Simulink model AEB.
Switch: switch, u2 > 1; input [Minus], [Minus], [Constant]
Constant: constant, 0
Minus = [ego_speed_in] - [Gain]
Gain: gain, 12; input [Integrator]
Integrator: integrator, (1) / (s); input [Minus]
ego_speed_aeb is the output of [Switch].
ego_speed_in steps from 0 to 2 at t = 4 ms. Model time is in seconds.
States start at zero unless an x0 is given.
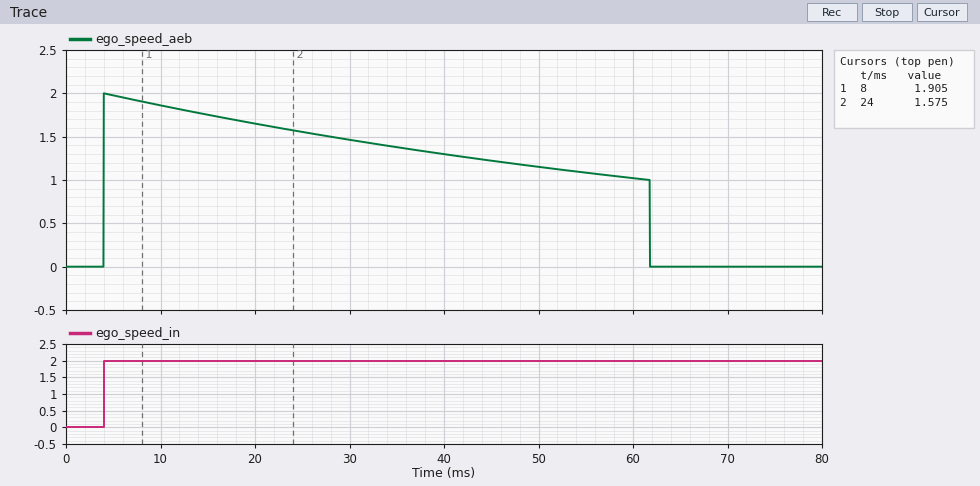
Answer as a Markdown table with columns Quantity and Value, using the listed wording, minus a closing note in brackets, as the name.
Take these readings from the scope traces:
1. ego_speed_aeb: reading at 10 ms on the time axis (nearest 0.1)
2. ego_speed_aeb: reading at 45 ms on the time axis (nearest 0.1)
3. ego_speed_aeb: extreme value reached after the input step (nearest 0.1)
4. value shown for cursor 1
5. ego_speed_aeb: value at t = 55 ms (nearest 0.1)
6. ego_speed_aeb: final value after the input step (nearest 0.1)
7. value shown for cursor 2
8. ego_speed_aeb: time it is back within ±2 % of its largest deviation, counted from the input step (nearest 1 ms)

| Quantity | Value |
|---|---|
| ego_speed_aeb: reading at 10 ms on the time axis | 1.9 |
| ego_speed_aeb: reading at 45 ms on the time axis | 1.2 |
| ego_speed_aeb: extreme value reached after the input step | 2.0 |
| value shown for cursor 1 | 1.905 |
| ego_speed_aeb: value at t = 55 ms | 1.1 |
| ego_speed_aeb: final value after the input step | 0.0 |
| value shown for cursor 2 | 1.575 |
| ego_speed_aeb: time it is back within ±2 % of its largest deviation, counted from the input step | 58 ms |
